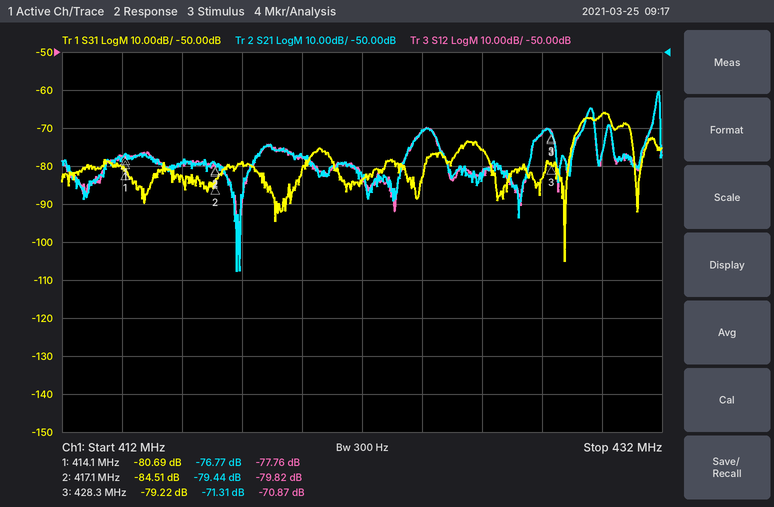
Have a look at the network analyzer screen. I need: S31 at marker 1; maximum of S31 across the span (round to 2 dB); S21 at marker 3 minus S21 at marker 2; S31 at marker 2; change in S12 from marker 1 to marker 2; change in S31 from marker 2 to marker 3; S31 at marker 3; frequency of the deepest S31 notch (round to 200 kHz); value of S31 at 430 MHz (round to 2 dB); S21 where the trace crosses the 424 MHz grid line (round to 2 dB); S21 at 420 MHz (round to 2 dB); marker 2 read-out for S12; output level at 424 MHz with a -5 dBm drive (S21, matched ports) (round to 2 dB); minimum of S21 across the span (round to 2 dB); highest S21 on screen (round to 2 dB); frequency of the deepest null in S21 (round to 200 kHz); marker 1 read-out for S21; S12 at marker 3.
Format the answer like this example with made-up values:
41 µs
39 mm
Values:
-80.69 dB
-66 dB
8.13 dB
-84.51 dB
-2.06 dB
5.29 dB
-79.22 dB
428.8 MHz
-66 dB
-70 dB
-78 dB
-79.82 dB
-76 dBm
-108 dB
-60 dB
417.8 MHz
-76.77 dB
-70.87 dB
